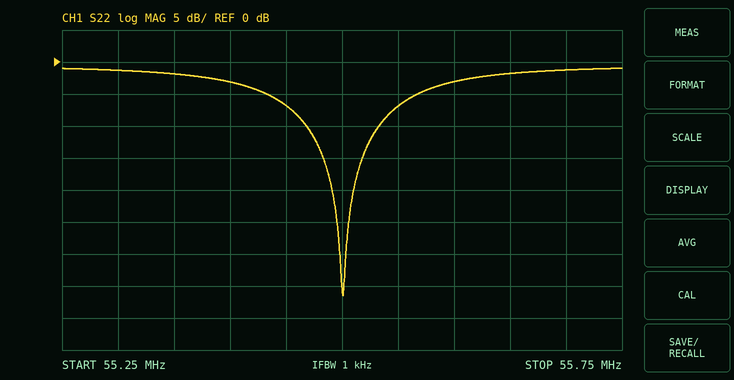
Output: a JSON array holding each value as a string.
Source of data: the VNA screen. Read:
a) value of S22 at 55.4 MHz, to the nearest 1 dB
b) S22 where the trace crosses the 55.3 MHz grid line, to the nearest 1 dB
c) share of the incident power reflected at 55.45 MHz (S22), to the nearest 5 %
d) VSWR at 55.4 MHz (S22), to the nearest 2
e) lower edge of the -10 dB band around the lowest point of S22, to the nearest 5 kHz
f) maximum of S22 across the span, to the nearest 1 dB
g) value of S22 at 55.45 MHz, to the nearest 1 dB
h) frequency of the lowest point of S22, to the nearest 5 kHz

["-3 dB", "-1 dB", "20 %", "6", "55.470 MHz", "-1 dB", "-7 dB", "55.500 MHz"]
